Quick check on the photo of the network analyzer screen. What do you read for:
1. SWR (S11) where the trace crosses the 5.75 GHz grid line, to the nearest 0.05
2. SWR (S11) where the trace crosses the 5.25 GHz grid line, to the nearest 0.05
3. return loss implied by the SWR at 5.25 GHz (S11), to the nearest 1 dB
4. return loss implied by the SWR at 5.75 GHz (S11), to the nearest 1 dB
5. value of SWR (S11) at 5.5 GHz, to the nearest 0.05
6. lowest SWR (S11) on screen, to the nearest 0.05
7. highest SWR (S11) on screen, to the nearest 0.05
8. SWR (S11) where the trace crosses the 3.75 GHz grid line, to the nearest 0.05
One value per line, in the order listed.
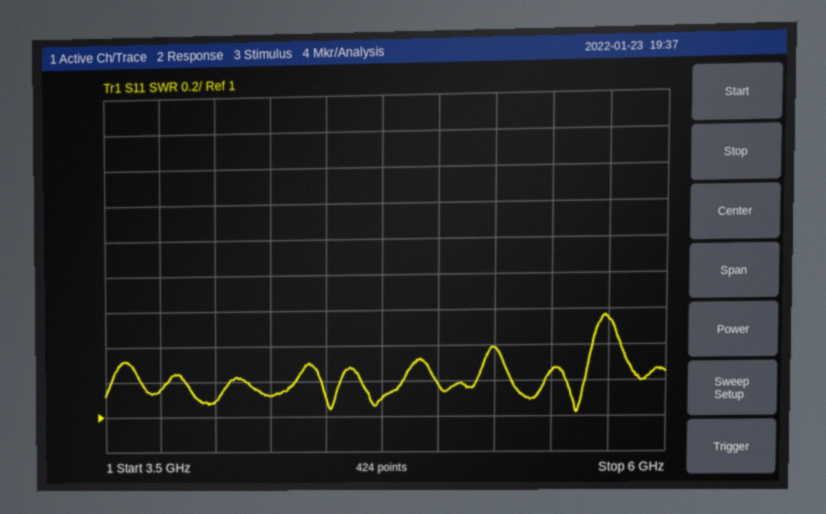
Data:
1.55
1.40
16 dB
13 dB
1.25
1.00
1.55
1.15
